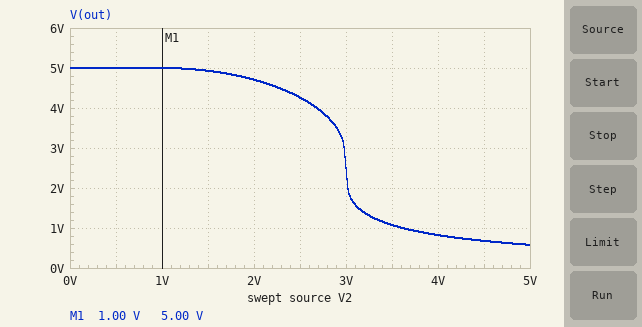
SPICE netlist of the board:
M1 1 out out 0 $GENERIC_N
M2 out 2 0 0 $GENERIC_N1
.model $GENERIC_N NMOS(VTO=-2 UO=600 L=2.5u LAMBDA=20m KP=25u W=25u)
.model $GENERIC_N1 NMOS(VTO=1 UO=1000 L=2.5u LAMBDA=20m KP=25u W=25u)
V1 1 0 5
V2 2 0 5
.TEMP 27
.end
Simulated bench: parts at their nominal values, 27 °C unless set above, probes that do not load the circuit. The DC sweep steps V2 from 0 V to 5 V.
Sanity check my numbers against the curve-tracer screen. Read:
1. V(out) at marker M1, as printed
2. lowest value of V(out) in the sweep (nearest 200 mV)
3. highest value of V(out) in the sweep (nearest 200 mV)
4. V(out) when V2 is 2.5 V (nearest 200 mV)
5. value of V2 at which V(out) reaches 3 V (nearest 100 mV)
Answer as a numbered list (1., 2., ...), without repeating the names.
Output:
1. 5.00 V
2. 600 mV
3. 5.0 V
4. 4.2 V
5. 3.0 V
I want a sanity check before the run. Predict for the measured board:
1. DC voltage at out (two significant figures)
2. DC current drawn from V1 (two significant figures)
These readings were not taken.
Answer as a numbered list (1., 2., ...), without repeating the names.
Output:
1. 580 mV
2. 540 µA
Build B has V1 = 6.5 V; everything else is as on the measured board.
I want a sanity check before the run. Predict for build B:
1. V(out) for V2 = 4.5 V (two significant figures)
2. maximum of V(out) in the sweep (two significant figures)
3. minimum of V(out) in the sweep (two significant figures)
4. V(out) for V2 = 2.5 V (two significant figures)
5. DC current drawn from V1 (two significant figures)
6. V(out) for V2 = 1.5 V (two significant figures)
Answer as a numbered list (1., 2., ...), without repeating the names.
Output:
1. 700 mV
2. 6.5 V
3. 600 mV
4. 5.7 V
5. 560 µA
6. 6.4 V
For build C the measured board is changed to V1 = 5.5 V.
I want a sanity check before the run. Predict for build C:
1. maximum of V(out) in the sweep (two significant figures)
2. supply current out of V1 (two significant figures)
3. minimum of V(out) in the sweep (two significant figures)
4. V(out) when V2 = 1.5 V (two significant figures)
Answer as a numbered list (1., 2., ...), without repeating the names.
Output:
1. 5.5 V
2. 550 µA
3. 590 mV
4. 5.4 V
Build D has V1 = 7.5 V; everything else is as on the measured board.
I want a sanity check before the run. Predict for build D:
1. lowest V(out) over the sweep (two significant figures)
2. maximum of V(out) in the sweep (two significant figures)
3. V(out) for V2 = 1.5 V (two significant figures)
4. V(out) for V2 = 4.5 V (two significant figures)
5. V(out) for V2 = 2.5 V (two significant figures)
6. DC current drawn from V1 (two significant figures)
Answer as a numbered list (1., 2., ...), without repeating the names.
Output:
1. 610 mV
2. 7.5 V
3. 7.4 V
4. 710 mV
5. 6.7 V
6. 570 µA
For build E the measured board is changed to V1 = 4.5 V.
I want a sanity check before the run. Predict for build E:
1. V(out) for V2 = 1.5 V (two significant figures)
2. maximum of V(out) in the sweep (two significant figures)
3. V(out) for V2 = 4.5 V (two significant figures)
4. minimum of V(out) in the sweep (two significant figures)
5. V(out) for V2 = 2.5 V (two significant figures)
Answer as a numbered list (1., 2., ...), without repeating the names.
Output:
1. 4.4 V
2. 4.5 V
3. 670 mV
4. 570 mV
5. 3.8 V
